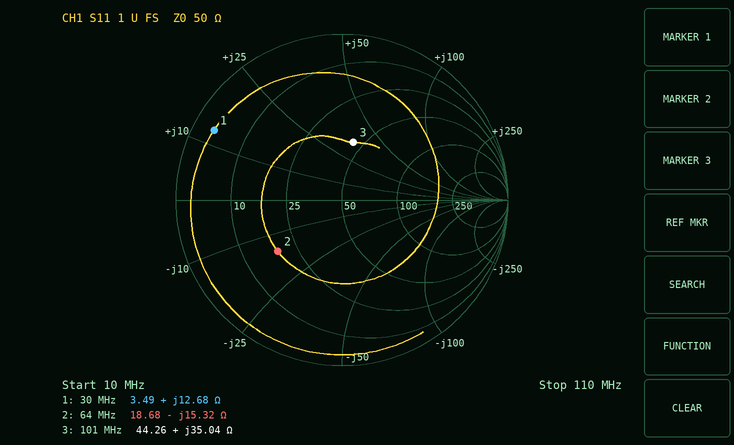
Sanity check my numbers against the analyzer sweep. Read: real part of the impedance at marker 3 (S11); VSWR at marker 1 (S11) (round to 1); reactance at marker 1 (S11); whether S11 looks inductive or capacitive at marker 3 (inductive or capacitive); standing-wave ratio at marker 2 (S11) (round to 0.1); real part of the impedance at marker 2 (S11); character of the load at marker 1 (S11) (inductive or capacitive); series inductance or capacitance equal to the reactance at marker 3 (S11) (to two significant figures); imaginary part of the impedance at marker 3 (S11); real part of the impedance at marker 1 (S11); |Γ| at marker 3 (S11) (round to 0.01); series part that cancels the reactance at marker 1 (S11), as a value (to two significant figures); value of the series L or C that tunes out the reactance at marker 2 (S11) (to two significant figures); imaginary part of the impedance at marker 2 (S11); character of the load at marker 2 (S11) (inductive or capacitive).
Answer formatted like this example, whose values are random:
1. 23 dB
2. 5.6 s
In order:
1. 44.26 Ω
2. 15
3. +12.68 Ω
4. inductive
5. 3.0
6. 18.68 Ω
7. inductive
8. 55 nH
9. +35.04 Ω
10. 3.49 Ω
11. 0.35
12. 420 pF
13. 38 nH
14. -15.32 Ω
15. capacitive
